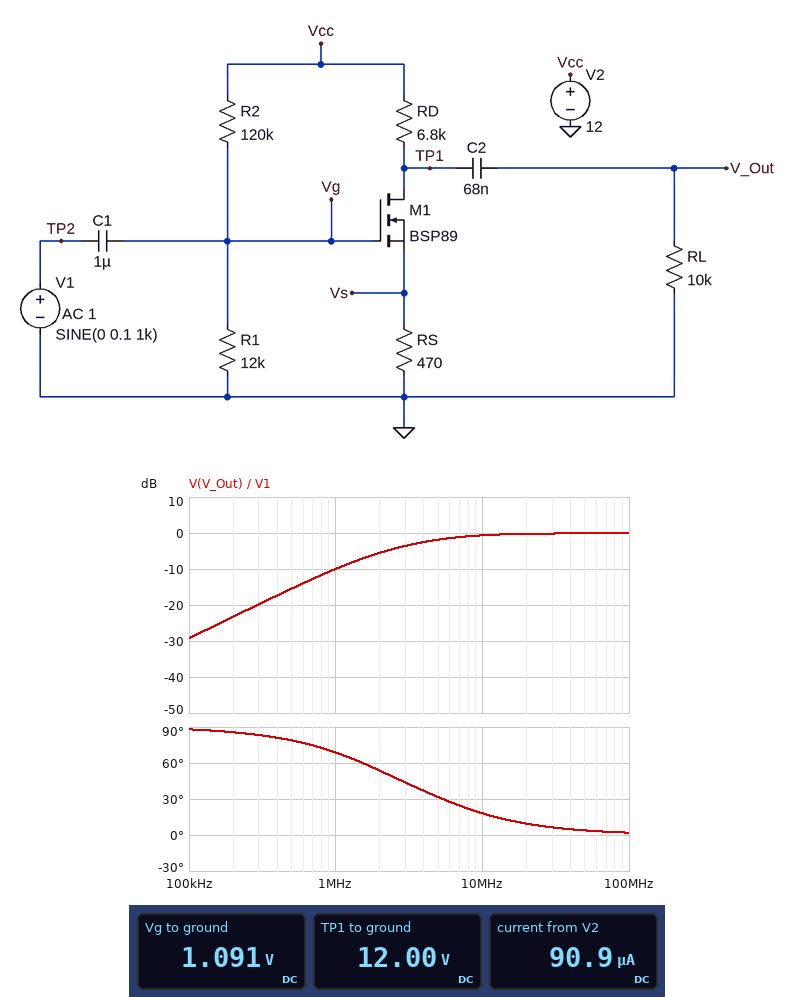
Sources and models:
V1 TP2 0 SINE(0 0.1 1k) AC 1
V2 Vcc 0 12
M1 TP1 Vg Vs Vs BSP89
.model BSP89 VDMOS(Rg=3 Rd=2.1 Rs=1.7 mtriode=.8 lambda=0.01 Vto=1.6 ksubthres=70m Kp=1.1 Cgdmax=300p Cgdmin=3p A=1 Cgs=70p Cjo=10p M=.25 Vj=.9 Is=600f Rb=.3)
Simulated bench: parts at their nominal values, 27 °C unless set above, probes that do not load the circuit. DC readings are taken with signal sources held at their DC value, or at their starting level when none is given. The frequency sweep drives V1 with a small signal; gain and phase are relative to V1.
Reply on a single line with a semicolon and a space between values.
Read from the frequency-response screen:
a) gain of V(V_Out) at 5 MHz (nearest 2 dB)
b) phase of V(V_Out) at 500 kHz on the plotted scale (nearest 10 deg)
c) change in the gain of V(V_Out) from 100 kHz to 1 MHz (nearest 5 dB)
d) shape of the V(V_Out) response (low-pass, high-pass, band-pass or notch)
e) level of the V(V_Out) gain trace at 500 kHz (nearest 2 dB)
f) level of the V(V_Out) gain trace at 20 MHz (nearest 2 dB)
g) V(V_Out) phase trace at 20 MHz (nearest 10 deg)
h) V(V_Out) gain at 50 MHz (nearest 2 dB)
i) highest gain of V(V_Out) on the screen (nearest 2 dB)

-2 dB; 80 deg; 20 dB; high-pass; -16 dB; 0 dB; 10 deg; 0 dB; 0 dB
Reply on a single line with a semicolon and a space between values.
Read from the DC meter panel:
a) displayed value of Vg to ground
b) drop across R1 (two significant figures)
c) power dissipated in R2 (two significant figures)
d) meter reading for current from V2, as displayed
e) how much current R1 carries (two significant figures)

1.091 V; 1.1 V; 990 µW; 90.9 µA; 91 µA
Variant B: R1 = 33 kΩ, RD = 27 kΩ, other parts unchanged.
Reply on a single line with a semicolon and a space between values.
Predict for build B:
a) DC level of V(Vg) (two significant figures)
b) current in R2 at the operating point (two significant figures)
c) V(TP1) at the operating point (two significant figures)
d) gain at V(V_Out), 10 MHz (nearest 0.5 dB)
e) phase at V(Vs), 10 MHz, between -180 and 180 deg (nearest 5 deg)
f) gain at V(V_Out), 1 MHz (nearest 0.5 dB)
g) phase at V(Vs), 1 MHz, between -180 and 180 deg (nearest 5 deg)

2.6 V; 78 µA; 210 mV; 0 dB; 5 deg; -3.0 dB; 45 deg
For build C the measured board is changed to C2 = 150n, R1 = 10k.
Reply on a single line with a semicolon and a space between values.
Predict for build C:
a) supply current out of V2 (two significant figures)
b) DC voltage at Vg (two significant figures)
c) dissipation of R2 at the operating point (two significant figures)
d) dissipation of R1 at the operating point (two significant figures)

92 µA; 920 mV; 1.0 mW; 85 µW
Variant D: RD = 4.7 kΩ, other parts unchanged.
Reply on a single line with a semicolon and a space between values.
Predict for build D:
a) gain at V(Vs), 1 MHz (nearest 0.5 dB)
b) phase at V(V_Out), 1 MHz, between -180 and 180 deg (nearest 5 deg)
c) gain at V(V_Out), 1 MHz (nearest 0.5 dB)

-14.0 dB; 75 deg; -11.5 dB
